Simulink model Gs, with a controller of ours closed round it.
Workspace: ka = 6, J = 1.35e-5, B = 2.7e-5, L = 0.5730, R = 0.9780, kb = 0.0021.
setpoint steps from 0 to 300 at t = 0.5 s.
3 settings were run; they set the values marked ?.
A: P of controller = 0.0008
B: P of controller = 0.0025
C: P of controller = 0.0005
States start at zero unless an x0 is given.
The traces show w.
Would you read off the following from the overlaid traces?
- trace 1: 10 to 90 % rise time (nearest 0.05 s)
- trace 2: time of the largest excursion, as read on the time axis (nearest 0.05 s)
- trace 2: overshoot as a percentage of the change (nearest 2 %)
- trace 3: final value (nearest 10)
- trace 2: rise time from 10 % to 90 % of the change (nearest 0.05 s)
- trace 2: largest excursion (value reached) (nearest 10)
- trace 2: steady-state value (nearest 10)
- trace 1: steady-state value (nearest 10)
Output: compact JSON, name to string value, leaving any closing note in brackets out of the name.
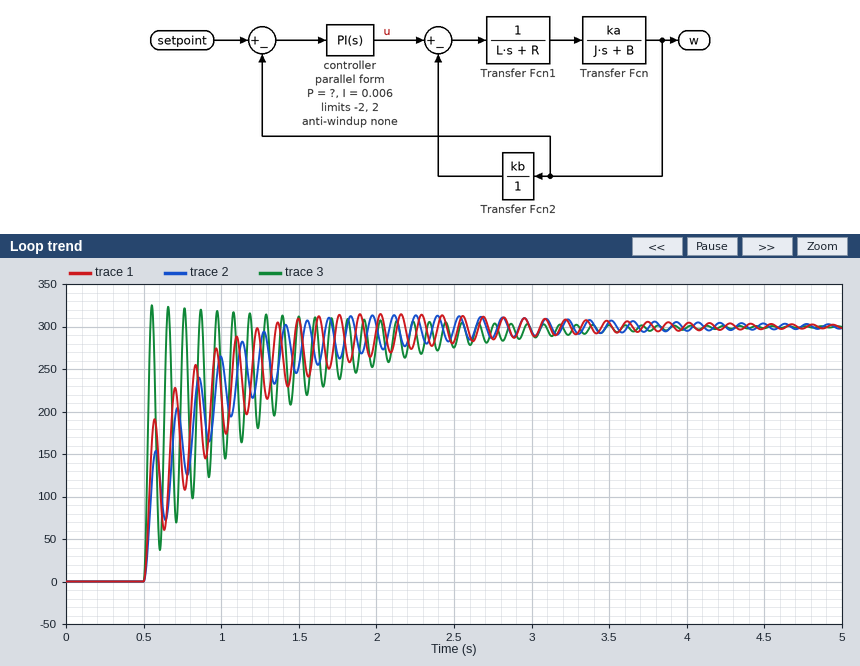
{"trace 1: 10 to 90 % rise time": "0.45 s", "trace 2: time of the largest excursion, as read on the time axis": "2.10 s", "trace 2: overshoot as a percentage of the change": "4 %", "trace 3: final value": "300", "trace 2: rise time from 10 % to 90 % of the change": "0.60 s", "trace 2: largest excursion (value reached)": "310", "trace 2: steady-state value": "300", "trace 1: steady-state value": "300"}
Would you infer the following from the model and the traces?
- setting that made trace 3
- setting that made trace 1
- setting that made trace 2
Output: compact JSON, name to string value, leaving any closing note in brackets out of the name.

{"setting that made trace 3": "B", "setting that made trace 1": "A", "setting that made trace 2": "C"}
